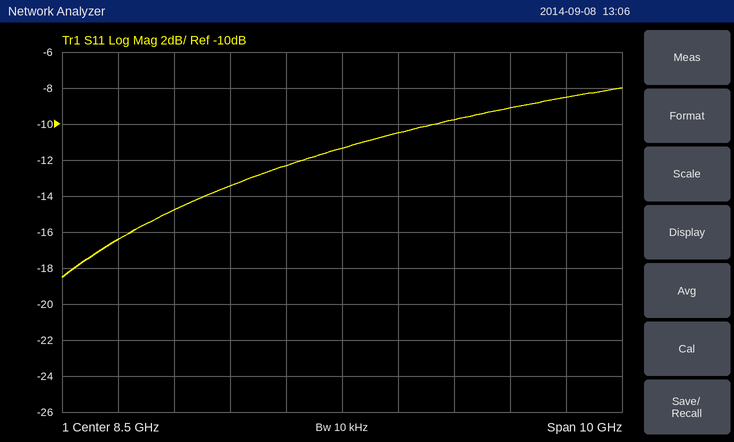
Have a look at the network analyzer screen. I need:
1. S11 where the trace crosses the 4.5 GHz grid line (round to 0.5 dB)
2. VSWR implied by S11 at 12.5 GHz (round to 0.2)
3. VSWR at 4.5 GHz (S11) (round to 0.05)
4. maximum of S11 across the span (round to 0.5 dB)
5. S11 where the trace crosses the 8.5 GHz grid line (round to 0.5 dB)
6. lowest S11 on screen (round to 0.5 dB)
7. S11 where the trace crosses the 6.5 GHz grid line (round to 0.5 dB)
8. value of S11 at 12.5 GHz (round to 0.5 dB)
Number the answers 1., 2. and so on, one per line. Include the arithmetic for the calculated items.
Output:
1. -16.5 dB
2. |Γ| = 10^(-8.5/20) = 0.3758; VSWR = (1 + 0.3758)/(1 − 0.3758) ≈ 2.2
3. |Γ| = 10^(-16.5/20) = 0.1496; VSWR = (1 + 0.1496)/(1 − 0.1496) ≈ 1.35
4. -8.0 dB
5. -11.5 dB
6. -18.5 dB
7. -13.5 dB
8. -8.5 dB
